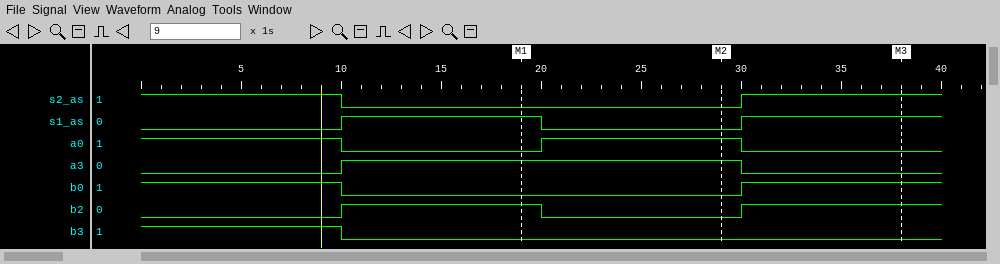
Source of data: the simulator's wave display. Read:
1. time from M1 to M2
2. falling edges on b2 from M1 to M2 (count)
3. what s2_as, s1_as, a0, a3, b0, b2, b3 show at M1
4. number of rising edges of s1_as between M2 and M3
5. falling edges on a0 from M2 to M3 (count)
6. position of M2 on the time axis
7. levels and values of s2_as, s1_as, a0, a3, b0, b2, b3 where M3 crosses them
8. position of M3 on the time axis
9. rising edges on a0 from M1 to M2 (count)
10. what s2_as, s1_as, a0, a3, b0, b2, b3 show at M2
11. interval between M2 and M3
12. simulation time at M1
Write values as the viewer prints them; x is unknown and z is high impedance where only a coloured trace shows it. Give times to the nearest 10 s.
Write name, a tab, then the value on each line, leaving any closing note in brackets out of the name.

time from M1 to M2	10 s
falling edges on b2 from M1 to M2	1
what s2_as, s1_as, a0, a3, b0, b2, b3 show at M1	s2_as=0, s1_as=1, a0=0, a3=1, b0=0, b2=1, b3=0
number of rising edges of s1_as between M2 and M3	1
falling edges on a0 from M2 to M3	1
position of M2 on the time axis	30 s
levels and values of s2_as, s1_as, a0, a3, b0, b2, b3 where M3 crosses them	s2_as=1, s1_as=1, a0=0, a3=0, b0=1, b2=1, b3=0
position of M3 on the time axis	40 s
rising edges on a0 from M1 to M2	1
what s2_as, s1_as, a0, a3, b0, b2, b3 show at M2	s2_as=0, s1_as=0, a0=1, a3=1, b0=0, b2=0, b3=0
interval between M2 and M3	10 s
simulation time at M1	20 s
